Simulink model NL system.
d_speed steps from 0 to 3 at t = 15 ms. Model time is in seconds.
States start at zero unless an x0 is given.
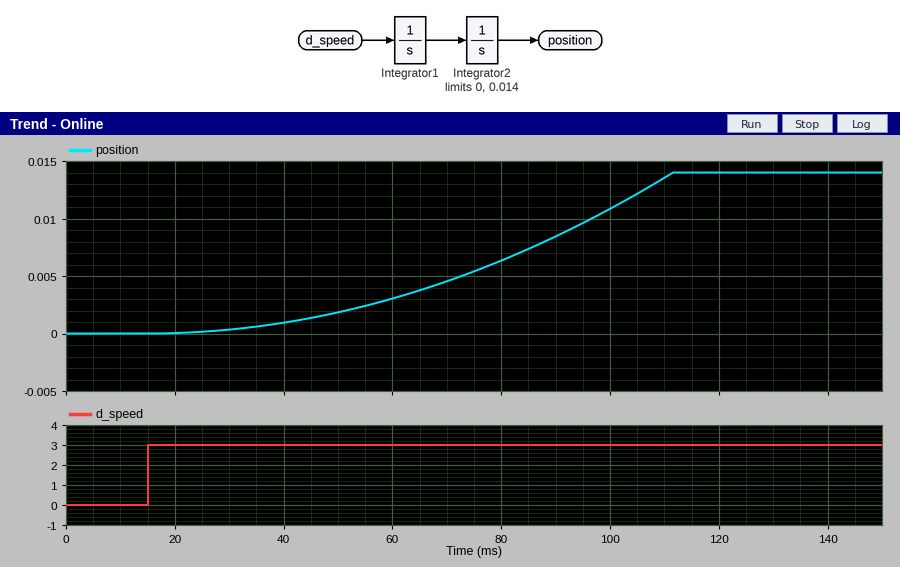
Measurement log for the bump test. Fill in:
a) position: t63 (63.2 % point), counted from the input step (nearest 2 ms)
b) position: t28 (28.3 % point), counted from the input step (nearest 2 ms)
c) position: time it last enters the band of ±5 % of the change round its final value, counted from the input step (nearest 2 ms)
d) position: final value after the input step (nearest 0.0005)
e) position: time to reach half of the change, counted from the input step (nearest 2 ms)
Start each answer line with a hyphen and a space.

- 76 ms
- 52 ms
- 94 ms
- 0.0140
- 68 ms
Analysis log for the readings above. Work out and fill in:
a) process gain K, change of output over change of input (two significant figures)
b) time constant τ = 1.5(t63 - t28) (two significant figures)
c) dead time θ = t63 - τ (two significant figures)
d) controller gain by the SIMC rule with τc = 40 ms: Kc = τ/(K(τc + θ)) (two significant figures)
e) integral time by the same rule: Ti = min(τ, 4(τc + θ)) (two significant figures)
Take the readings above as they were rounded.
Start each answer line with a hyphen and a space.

- 0.0047
- 36 ms
- 40 ms
- 96
- 36 ms
